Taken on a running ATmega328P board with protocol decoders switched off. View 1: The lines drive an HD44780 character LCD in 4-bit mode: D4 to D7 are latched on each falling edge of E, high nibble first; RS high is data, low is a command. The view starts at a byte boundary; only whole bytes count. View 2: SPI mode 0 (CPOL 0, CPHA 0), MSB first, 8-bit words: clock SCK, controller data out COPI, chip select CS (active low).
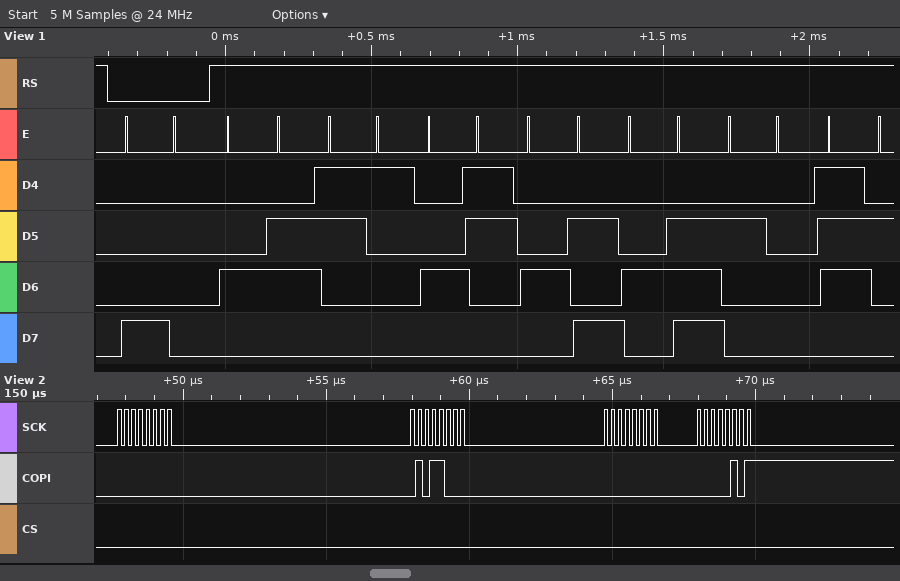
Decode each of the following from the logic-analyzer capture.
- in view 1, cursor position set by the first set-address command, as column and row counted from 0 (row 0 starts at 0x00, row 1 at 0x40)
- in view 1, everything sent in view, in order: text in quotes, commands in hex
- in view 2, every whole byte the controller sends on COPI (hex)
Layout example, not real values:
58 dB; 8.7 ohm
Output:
column 0, row 0; 0x80 "F1CJN r"; 00 58 00 05
